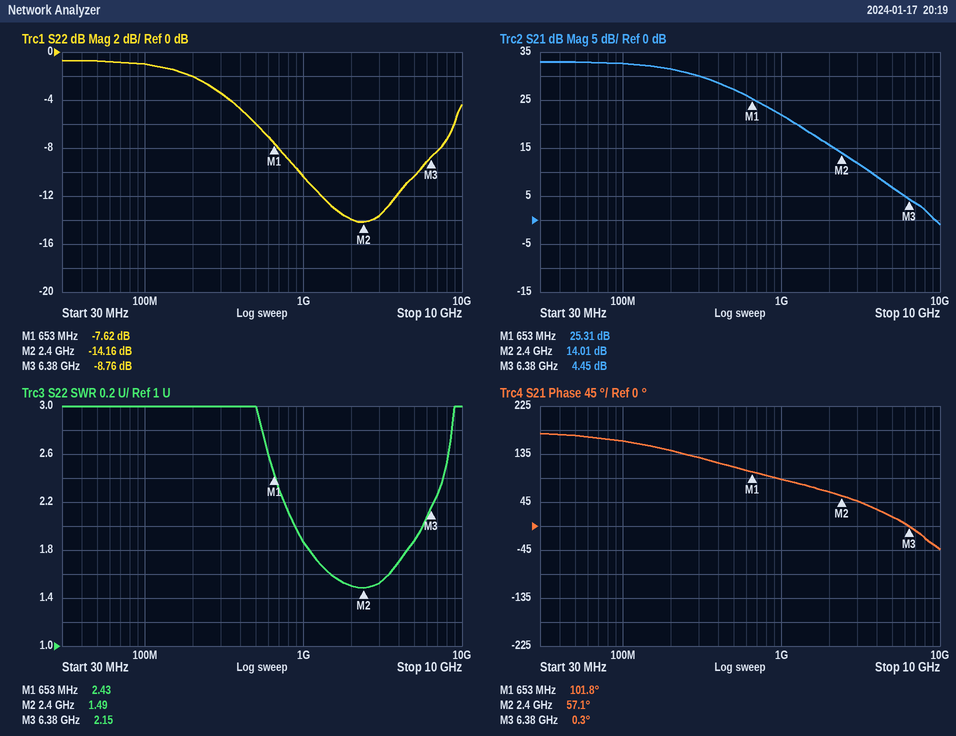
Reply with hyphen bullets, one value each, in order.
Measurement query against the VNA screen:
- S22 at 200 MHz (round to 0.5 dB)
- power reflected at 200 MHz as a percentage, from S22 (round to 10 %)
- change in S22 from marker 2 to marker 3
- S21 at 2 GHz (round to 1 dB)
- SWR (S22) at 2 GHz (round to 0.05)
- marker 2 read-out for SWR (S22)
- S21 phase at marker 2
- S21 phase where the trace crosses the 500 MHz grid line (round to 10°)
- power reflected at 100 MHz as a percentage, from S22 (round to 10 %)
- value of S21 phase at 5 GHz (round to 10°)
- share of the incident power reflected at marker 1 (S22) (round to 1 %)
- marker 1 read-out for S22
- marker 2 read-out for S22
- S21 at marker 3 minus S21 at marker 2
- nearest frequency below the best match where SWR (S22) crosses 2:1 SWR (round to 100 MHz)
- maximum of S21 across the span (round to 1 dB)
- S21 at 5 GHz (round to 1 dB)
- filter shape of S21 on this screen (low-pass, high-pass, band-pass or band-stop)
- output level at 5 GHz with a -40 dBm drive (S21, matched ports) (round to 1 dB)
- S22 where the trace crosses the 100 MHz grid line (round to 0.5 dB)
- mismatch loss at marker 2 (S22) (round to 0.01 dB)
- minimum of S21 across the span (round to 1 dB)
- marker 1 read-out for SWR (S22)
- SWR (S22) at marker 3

- -2.0 dB
- 60 %
- 5.40 dB
- 16 dB
- 1.50
- 1.49
- 57.1°
- 110°
- 80 %
- 20°
- 17 %
- -7.62 dB
- -14.16 dB
- -9.56 dB
- 900 MHz
- 33 dB
- 7 dB
- low-pass
- -33 dBm
- -1.0 dB
- 0.17 dB
- -1 dB
- 2.43
- 2.15
